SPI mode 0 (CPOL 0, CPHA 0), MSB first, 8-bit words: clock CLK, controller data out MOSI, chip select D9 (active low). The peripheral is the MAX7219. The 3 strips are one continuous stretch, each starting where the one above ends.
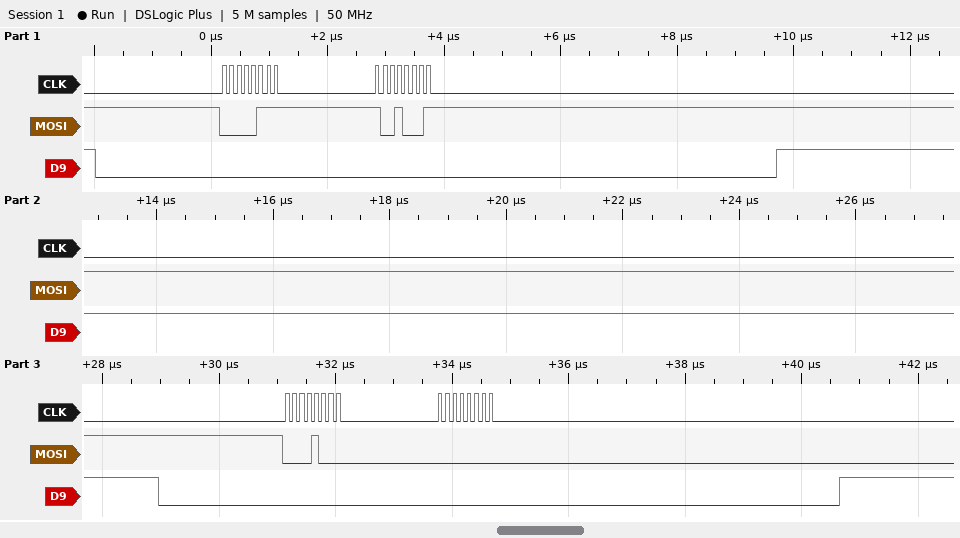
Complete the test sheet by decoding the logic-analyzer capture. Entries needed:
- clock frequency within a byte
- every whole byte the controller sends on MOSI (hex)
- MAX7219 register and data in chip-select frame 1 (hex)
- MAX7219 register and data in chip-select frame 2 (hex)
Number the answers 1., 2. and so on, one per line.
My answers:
1. 8 MHz
2. 07 91 08 00
3. register 0x7, data 0x91
4. register 0x8, data 0x00
